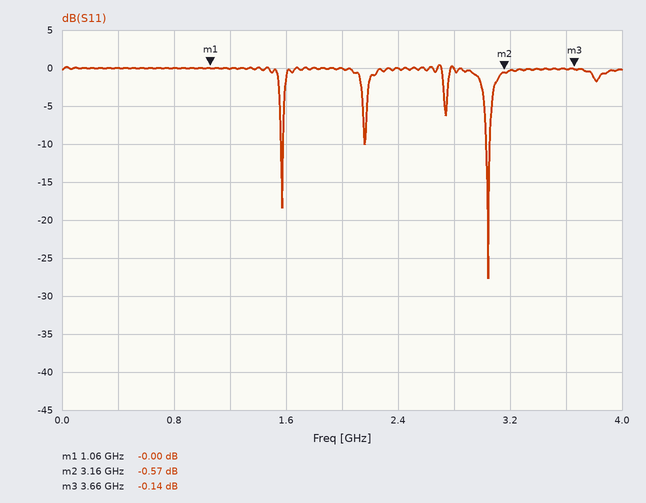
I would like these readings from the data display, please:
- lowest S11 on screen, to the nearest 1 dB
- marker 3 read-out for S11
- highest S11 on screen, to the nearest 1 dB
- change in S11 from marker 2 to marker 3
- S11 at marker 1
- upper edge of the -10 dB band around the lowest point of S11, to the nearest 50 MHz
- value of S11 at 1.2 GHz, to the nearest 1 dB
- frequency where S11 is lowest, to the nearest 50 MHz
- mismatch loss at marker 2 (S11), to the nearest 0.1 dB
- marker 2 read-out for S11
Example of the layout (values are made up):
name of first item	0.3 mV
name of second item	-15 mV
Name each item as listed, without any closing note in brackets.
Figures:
lowest S11 on screen, to the nearest 1 dB	-28 dB
marker 3 read-out for S11	-0.14 dB
highest S11 on screen, to the nearest 1 dB	0 dB
change in S11 from marker 2 to marker 3	0.43 dB
S11 at marker 1	-0.00 dB
upper edge of the -10 dB band around the lowest point of S11, to the nearest 50 MHz	3.05 GHz
value of S11 at 1.2 GHz, to the nearest 1 dB	0 dB
frequency where S11 is lowest, to the nearest 50 MHz	3.05 GHz
mismatch loss at marker 2 (S11), to the nearest 0.1 dB	9.1 dB
marker 2 read-out for S11	-0.57 dB
